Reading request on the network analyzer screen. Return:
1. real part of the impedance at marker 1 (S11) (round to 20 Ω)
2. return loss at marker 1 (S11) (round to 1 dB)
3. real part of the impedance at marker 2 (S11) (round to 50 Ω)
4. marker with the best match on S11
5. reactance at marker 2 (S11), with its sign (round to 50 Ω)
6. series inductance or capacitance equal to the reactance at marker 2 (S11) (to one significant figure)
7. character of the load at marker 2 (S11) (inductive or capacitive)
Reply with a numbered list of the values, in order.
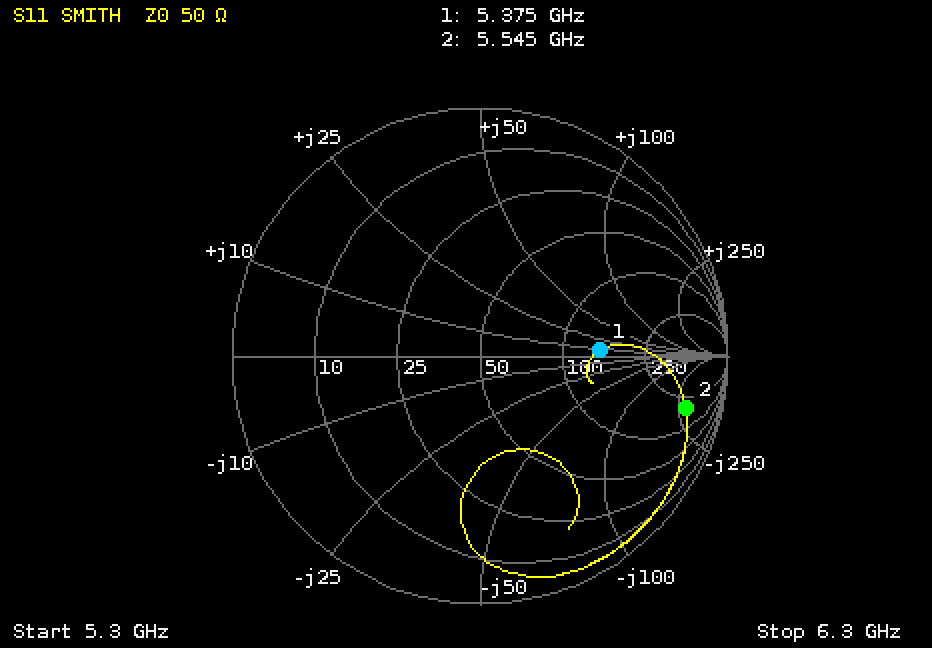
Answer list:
1. 140 Ω
2. 6 dB
3. 200 Ω
4. marker 1
5. -300 Ω
6. 100 fF
7. capacitive
